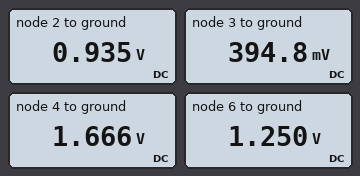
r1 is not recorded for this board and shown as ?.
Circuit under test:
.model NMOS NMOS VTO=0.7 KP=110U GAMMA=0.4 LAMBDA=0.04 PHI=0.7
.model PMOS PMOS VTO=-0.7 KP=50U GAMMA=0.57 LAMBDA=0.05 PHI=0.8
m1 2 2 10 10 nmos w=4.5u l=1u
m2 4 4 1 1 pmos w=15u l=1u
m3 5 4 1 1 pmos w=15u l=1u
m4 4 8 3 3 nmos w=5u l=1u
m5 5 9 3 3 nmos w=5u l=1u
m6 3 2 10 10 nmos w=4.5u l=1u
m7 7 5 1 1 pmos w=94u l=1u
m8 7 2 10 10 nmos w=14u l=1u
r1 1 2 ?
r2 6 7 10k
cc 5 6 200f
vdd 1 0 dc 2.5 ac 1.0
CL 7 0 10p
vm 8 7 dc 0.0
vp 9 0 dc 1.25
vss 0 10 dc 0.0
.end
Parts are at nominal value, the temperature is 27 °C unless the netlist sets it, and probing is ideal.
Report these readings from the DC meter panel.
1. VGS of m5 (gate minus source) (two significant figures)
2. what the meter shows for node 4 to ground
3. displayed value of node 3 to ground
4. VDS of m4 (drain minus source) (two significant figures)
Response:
860 mV
1.666 V
394.8 mV
1.3 V
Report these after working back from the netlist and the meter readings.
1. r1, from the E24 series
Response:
110 kΩ
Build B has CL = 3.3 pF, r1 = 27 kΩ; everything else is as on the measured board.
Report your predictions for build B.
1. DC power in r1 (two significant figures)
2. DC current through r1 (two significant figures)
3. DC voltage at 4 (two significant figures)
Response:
68 µW
50 µA
1.6 V
